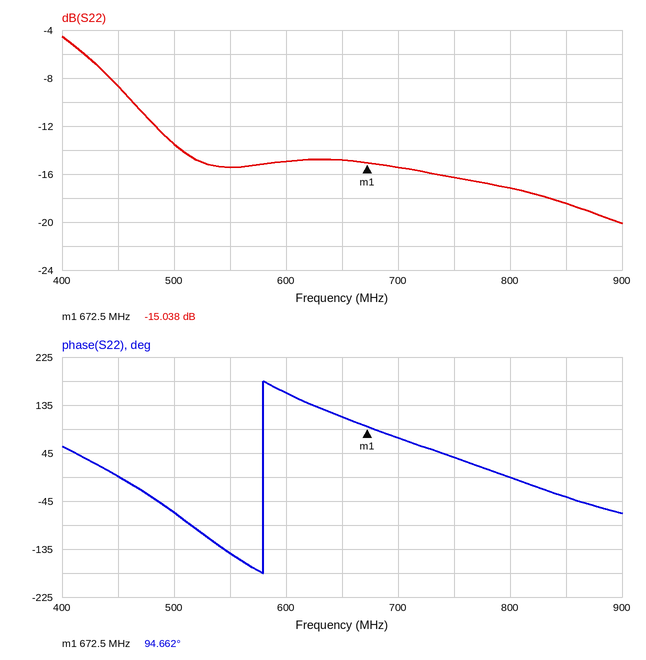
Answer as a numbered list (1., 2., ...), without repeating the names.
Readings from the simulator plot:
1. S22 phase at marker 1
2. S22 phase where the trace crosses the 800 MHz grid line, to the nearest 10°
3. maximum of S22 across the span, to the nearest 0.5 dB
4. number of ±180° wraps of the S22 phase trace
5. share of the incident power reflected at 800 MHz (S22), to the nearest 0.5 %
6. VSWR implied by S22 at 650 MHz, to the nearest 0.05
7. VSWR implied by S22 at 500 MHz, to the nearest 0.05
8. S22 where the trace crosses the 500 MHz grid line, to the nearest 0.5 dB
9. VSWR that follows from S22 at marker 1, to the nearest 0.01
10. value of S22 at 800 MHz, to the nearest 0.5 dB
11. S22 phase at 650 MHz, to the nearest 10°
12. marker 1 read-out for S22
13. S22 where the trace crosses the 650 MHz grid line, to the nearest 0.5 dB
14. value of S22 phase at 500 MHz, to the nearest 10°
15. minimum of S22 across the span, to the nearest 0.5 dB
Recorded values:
1. 94.662°
2. 0°
3. -4.5 dB
4. 1
5. 2.0 %
6. 1.45
7. 1.55
8. -13.5 dB
9. 1.43
10. -17.0 dB
11. 110°
12. -15.038 dB
13. -15.0 dB
14. -70°
15. -20.0 dB
